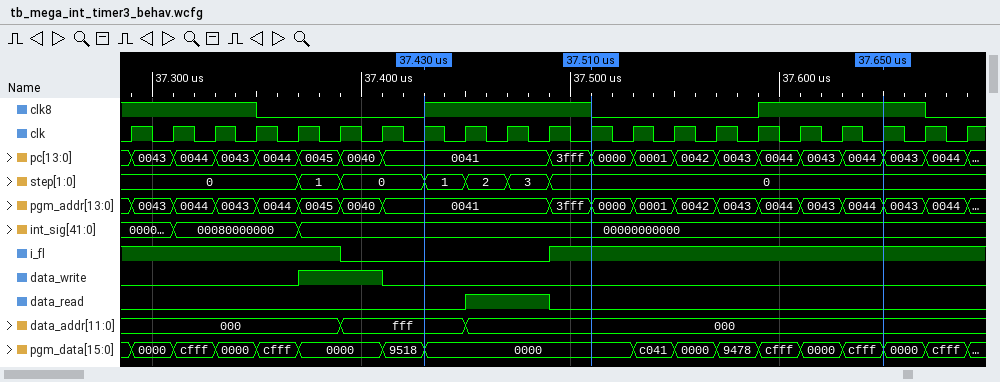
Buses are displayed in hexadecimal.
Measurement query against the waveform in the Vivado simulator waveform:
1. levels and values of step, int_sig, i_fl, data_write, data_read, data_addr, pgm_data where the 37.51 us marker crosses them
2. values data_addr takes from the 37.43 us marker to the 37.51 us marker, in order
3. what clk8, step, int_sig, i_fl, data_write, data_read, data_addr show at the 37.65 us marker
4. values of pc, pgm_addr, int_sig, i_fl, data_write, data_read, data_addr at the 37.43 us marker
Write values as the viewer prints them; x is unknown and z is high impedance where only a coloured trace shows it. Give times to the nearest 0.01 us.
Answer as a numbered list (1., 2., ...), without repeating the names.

1. step=0, int_sig=00000000000, i_fl=1, data_write=0, data_read=0, data_addr=000, pgm_data=0000
2. fff, 000
3. clk8=1, step=0, int_sig=00000000000, i_fl=1, data_write=0, data_read=0, data_addr=000
4. pc=0041, pgm_addr=0041, int_sig=00000000000, i_fl=0, data_write=0, data_read=0, data_addr=fff
